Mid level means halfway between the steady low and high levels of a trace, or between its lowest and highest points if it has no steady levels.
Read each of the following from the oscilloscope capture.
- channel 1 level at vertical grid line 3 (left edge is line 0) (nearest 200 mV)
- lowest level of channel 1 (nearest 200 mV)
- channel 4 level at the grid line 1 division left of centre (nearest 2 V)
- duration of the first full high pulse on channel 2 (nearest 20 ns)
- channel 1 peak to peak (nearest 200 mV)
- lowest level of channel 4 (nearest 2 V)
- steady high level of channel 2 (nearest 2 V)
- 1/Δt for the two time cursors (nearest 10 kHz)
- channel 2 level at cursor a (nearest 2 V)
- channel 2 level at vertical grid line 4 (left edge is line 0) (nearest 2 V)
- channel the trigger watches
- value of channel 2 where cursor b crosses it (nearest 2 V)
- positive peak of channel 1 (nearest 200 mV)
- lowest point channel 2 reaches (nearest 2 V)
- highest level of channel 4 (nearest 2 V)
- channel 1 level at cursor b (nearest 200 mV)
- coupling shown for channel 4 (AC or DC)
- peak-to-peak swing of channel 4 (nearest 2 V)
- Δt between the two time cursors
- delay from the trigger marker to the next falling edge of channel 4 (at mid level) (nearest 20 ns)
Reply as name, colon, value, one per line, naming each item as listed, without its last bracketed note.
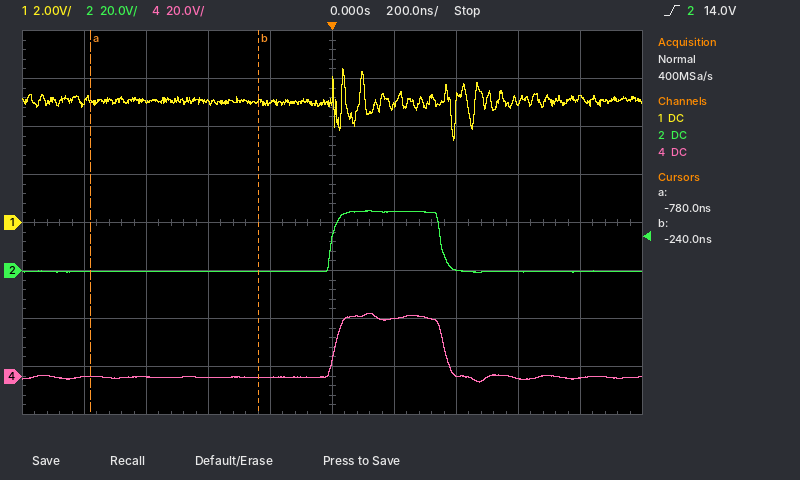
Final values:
channel 1 level at vertical grid line 3 (left edge is line 0): 5.0 V
lowest level of channel 1: 3.4 V
channel 4 level at the grid line 1 division left of centre: 0 V
duration of the first full high pulse on channel 2: 360 ns
channel 1 peak to peak: 3.0 V
lowest level of channel 4: -2 V
steady high level of channel 2: 24 V
1/Δt for the two time cursors: 1.85 MHz
channel 2 level at cursor a: 0 V
channel 2 level at vertical grid line 4 (left edge is line 0): 0 V
channel the trigger watches: channel 2
value of channel 2 where cursor b crosses it: 0 V
positive peak of channel 1: 6.4 V
lowest point channel 2 reaches: 0 V
highest level of channel 4: 26 V
channel 1 level at cursor b: 5.0 V
coupling shown for channel 4: DC
peak-to-peak swing of channel 4: 28 V
Δt between the two time cursors: 540 ns
delay from the trigger marker to the next falling edge of channel 4 (at mid level): 360 ns
